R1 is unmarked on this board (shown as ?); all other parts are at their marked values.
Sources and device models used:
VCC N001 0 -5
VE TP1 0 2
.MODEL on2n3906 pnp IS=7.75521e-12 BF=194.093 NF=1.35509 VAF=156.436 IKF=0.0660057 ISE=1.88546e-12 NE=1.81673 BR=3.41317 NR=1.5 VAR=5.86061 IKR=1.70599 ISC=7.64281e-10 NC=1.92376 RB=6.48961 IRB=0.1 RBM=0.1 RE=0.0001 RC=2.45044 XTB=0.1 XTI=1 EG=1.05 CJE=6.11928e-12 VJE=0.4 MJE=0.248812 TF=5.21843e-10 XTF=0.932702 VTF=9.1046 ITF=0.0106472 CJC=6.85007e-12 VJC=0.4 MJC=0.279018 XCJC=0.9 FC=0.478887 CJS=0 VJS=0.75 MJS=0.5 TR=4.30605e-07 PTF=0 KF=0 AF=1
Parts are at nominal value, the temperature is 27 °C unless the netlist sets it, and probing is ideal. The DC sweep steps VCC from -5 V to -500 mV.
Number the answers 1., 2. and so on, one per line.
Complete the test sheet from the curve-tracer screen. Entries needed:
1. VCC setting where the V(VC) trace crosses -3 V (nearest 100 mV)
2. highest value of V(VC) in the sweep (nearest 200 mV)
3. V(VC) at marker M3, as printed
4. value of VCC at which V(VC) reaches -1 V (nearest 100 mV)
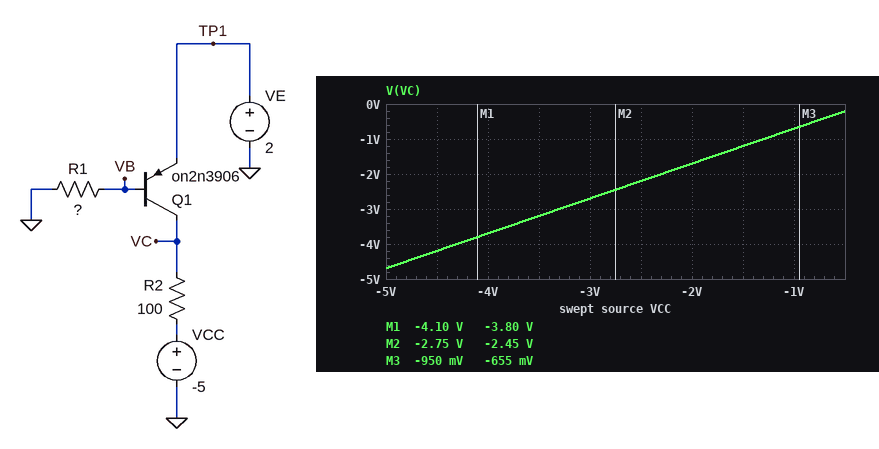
1. -3.3 V
2. -200 mV
3. -655 mV
4. -1.3 V
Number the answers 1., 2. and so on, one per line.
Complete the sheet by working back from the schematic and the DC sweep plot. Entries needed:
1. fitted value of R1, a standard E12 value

1. 56 kΩ
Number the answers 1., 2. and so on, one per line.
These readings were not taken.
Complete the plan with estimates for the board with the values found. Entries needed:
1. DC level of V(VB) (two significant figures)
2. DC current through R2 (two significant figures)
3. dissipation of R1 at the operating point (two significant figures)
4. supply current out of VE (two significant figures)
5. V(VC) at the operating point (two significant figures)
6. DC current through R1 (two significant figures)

1. 1.3 V
2. 3.0 mA
3. 30 µW
4. 3.1 mA
5. -4.7 V
6. 23 µA
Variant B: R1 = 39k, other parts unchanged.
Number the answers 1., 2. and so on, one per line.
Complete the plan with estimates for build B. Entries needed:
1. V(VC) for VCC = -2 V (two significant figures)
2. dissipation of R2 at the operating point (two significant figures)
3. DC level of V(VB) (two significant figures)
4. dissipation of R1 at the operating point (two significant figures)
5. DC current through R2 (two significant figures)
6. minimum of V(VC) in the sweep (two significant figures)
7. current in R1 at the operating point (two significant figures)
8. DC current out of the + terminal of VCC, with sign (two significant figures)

1. -1.6 V
2. 1.9 mW
3. 1.3 V
4. 43 µW
5. 4.3 mA
6. -4.6 V
7. 33 µA
8. -4.3 mA
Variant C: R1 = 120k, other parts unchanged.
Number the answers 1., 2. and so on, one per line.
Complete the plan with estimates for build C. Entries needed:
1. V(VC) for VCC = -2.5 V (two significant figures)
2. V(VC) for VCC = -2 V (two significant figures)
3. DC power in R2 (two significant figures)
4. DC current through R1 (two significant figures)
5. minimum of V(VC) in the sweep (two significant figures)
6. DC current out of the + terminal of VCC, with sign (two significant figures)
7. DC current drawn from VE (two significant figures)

1. -2.4 V
2. -1.9 V
3. 200 µW
4. 11 µA
5. -4.9 V
6. -1.4 mA
7. 1.4 mA
